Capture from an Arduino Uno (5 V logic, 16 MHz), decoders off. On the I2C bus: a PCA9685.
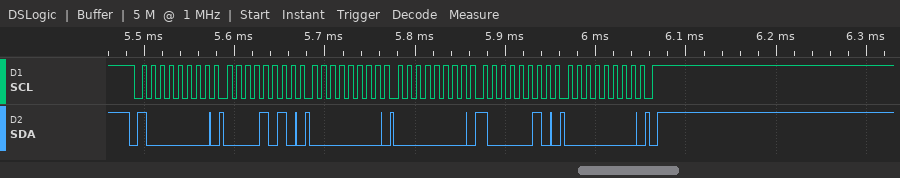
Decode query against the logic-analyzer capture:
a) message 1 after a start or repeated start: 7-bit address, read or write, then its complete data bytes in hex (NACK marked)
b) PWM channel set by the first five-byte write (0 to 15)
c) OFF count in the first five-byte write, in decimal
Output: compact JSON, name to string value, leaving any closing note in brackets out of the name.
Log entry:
{"message 1 after a start or repeated start: 7-bit address, read or write, then its complete data bytes in hex": "0x40 write: 0A 00 00 82 00", "PWM channel set by the first five-byte write": "1", "OFF count in the first five-byte write, in decimal": "130"}
